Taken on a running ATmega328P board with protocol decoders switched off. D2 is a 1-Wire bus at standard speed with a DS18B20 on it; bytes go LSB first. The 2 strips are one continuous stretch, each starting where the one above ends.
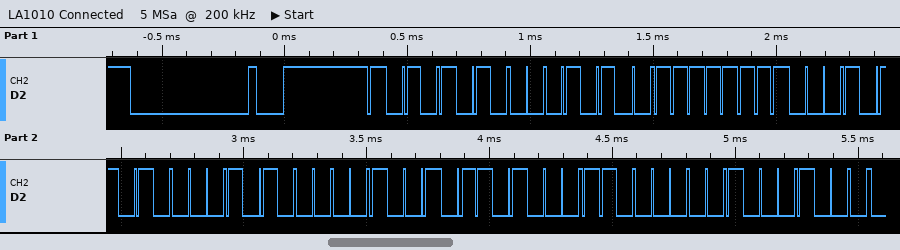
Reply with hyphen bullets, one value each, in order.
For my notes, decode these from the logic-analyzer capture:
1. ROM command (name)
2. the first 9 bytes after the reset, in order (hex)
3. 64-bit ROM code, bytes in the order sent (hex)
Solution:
- Match ROM
- 55 28 FF A8 50 90 16 03 11
- 28 FF A8 50 90 16 03 11
